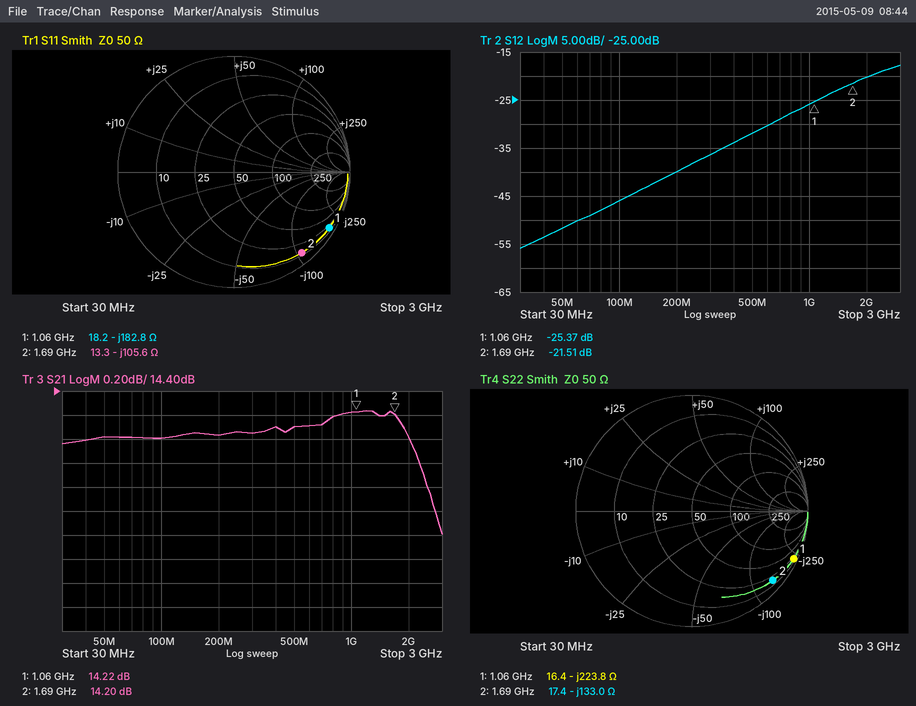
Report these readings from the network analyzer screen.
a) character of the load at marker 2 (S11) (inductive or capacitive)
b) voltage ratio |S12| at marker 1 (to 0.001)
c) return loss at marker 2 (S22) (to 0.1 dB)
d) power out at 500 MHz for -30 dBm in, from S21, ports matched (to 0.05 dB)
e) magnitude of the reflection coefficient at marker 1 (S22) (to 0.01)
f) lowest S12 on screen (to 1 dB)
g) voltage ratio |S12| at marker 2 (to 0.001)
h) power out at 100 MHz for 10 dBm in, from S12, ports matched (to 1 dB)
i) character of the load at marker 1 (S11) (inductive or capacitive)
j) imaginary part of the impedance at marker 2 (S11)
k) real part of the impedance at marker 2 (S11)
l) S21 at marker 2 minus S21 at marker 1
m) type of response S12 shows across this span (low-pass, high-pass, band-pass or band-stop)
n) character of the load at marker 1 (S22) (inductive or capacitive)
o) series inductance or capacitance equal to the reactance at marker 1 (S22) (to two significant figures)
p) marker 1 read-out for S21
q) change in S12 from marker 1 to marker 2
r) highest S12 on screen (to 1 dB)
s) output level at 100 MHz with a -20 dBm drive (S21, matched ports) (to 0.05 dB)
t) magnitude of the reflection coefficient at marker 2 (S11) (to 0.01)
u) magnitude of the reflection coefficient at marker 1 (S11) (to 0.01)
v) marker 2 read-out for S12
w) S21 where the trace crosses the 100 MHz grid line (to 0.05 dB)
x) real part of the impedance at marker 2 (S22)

capacitive
0.054
0.7 dB
-15.90 dBm
0.97
-56 dB
0.084
-36 dBm
capacitive
-105.6 Ω
13.3 Ω
-0.02 dB
high-pass
capacitive
670 fF
14.22 dB
3.86 dB
-18 dB
-6.00 dBm
0.91
0.95
-21.51 dB
14.00 dB
17.4 Ω
